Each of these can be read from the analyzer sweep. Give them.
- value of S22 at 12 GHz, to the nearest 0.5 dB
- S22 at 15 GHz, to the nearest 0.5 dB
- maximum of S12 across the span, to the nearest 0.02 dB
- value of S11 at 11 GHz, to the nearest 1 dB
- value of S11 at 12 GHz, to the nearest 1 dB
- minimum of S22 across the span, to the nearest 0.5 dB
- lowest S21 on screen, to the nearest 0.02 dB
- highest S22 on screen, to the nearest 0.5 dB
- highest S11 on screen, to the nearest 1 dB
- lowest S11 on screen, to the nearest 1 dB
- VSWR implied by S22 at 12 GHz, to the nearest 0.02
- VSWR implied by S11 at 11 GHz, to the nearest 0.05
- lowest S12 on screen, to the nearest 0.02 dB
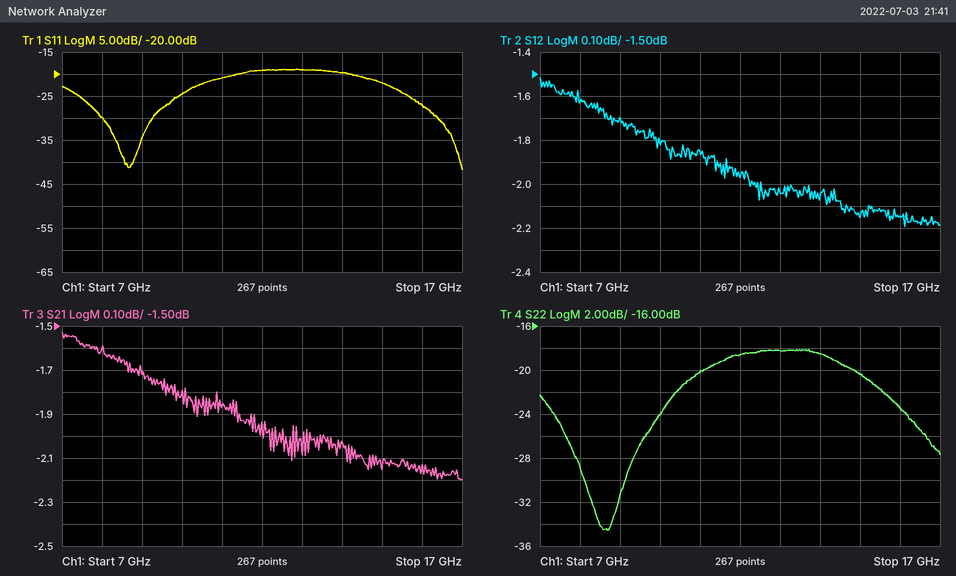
-18.5 dB
-20.5 dB
-1.52 dB
-21 dB
-19 dB
-34.5 dB
-2.20 dB
-18.0 dB
-19 dB
-42 dB
1.26
1.20
-2.20 dB
